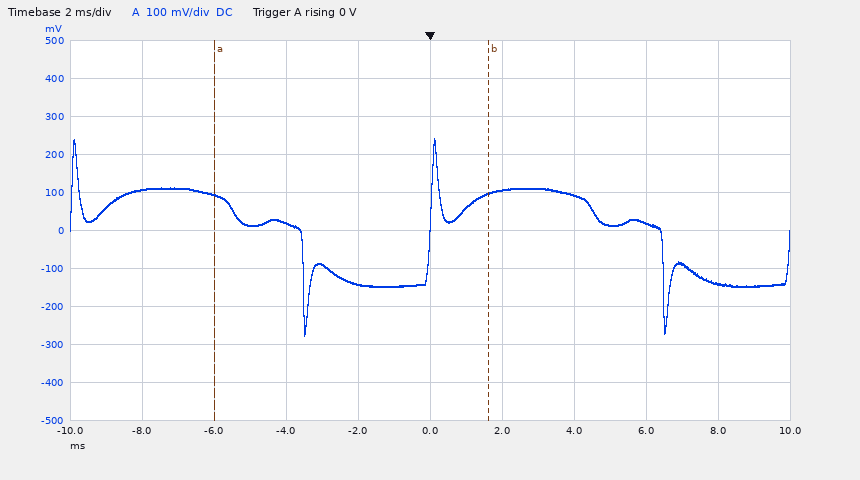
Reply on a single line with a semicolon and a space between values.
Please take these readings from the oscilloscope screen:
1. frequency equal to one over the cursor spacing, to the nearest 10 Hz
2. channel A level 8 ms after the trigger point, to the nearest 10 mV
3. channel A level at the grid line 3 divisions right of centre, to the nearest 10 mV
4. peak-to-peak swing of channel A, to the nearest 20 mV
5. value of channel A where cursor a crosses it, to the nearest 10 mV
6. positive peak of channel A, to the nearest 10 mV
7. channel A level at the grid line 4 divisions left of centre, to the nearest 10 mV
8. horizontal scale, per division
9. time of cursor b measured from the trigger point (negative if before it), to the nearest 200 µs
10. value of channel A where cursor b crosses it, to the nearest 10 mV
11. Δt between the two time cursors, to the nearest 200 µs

130 Hz; -140 mV; 20 mV; 520 mV; 90 mV; 240 mV; 110 mV; 2 ms; +1.6 ms; 100 mV; 7.6 ms
